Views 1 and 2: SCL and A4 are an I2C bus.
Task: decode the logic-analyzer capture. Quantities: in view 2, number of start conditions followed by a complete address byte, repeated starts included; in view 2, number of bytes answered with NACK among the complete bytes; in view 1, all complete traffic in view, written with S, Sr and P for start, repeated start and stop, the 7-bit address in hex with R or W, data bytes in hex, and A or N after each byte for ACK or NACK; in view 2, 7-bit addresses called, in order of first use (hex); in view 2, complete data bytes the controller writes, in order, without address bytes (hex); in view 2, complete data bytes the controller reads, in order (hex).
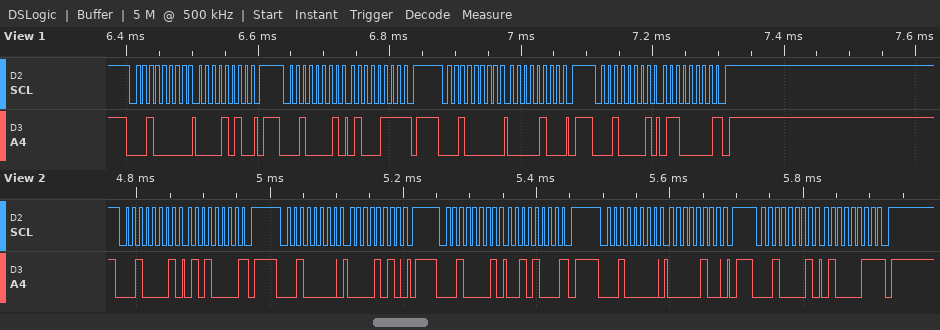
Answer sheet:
5
3
S 10W A 0A A P S 10R A 47 N P S 10W A 04 A P S 10R A 60 N P
0x10
0A 04
50 28 43
